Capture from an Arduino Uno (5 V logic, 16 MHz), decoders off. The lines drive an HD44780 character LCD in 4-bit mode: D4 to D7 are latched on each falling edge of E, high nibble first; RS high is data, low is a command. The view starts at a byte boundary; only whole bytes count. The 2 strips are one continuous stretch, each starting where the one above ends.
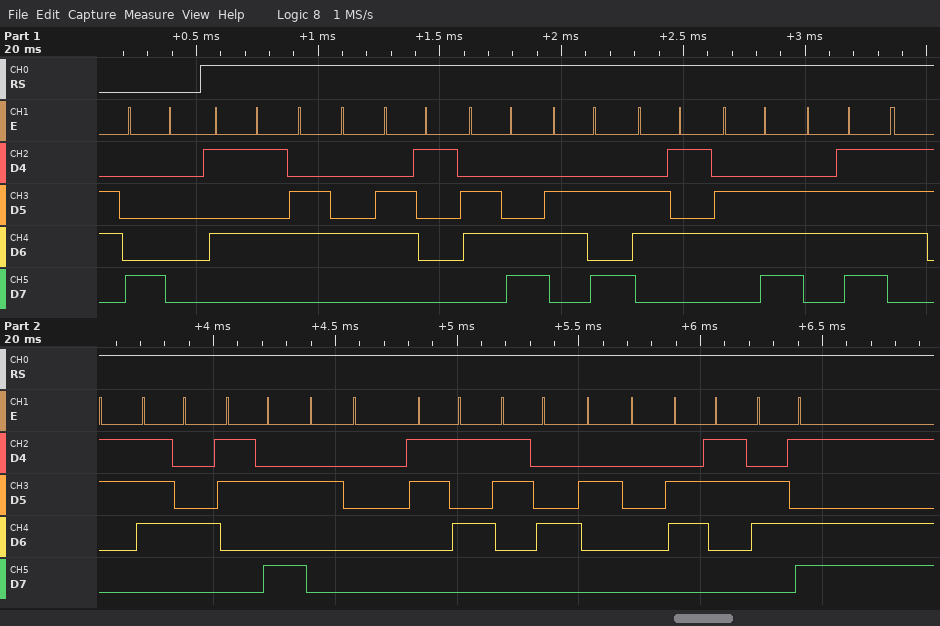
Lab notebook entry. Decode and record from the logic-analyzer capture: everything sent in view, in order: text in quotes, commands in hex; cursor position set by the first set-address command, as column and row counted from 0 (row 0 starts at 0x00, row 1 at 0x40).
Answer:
0x80 "Udaljenost: 54 cm"
column 0, row 0
